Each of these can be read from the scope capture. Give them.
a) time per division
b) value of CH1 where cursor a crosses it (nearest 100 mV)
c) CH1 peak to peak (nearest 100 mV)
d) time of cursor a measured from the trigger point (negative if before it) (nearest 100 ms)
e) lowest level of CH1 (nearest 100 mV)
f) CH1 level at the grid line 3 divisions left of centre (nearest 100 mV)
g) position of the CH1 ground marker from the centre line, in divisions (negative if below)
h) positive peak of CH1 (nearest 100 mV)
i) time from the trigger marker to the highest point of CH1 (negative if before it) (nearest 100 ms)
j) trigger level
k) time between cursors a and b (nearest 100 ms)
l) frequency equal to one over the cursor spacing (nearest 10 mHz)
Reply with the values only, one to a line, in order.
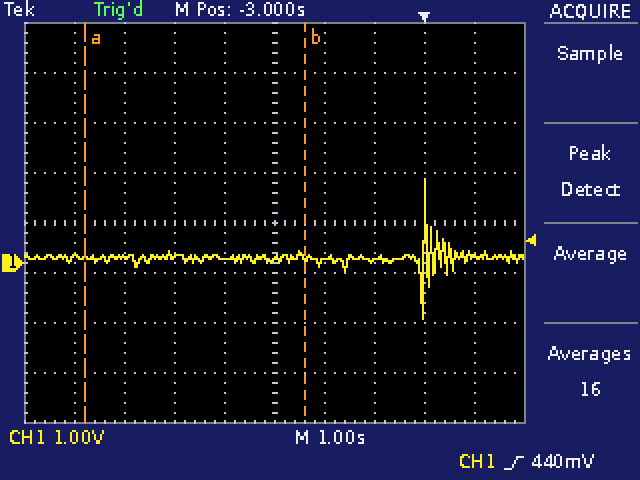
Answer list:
1 s
100 mV
2.8 V
-6.8 s
-1.1 V
100 mV
-0.8 div
1.7 V
0.0 s
440 mV
4.4 s
230 mHz
